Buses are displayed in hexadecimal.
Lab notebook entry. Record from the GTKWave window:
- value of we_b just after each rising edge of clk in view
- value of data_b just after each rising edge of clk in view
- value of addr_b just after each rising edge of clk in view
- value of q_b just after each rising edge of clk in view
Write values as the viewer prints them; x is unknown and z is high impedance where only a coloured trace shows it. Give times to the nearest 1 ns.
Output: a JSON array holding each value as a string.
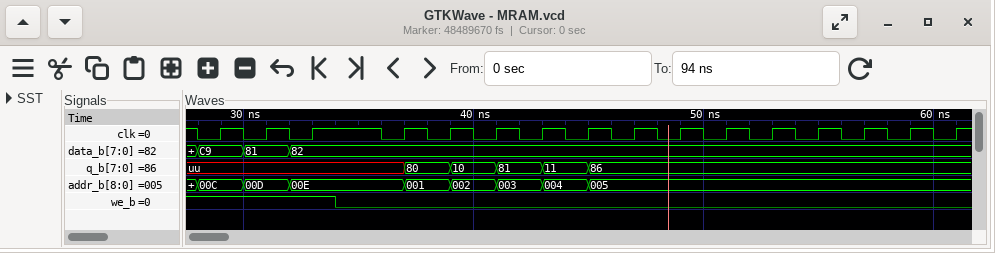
["1 1 1 0 0 0 0 0 0 0 0 0 0 0 0 0", "C9, 81, 82, 82, 82, 82, 82, 82, 82, 82, 82, 82, 82, 82, 82, 82", "00C, 00D, 00E, 001, 002, 003, 004, 005, 005, 005, 005, 005, 005, 005, 005, 005", "uu, uu, uu, 80, 10, 81, 11, 86, 86, 86, 86, 86, 86, 86, 86, 86"]
